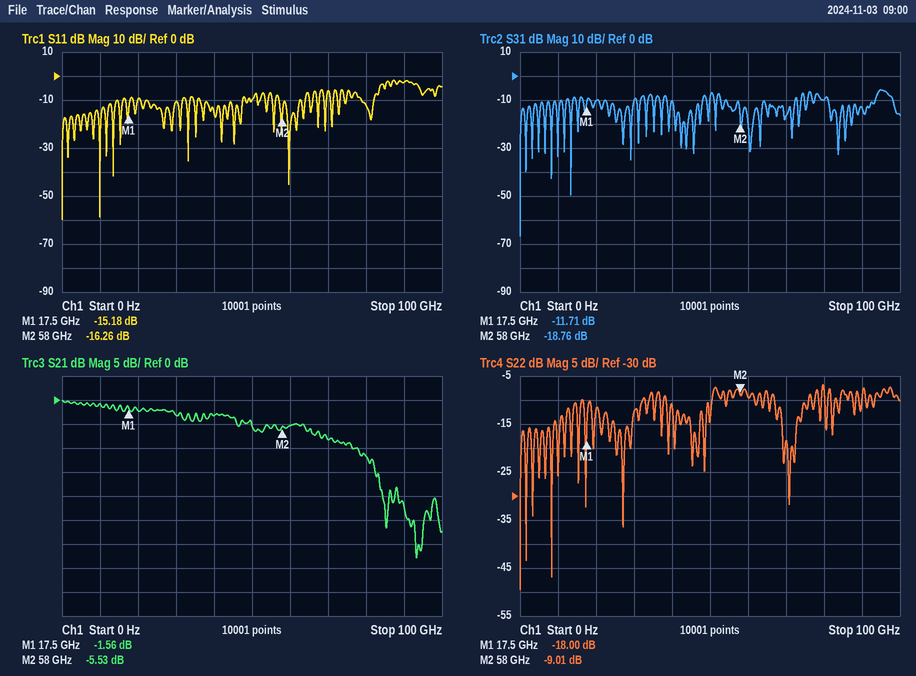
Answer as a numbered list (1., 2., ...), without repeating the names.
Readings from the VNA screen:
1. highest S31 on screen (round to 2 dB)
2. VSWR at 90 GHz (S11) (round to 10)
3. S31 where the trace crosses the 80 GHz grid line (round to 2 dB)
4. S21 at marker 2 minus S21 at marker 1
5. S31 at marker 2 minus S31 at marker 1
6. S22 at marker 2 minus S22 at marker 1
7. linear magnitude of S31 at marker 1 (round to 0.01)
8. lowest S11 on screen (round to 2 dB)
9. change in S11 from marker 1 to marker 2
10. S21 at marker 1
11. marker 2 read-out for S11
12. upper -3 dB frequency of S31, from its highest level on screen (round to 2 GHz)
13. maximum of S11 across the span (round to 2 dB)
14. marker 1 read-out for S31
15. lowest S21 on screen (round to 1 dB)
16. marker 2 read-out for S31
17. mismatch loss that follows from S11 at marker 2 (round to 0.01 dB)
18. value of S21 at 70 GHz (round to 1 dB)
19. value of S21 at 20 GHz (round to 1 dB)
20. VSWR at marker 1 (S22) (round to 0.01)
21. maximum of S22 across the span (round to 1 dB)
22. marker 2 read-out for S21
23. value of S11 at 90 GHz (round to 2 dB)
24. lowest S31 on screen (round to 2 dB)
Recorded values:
1. -6 dB
2. 10
3. -10 dB
4. -3.97 dB
5. -7.05 dB
6. 8.99 dB
7. 0.26
8. -60 dB
9. -1.08 dB
10. -1.56 dB
11. -16.26 dB
12. 98 GHz
13. -2 dB
14. -11.71 dB
15. -33 dB
16. -18.76 dB
17. 0.10 dB
18. -8 dB
19. -2 dB
20. 1.29
21. -7 dB
22. -5.53 dB
23. -2 dB
24. -66 dB
